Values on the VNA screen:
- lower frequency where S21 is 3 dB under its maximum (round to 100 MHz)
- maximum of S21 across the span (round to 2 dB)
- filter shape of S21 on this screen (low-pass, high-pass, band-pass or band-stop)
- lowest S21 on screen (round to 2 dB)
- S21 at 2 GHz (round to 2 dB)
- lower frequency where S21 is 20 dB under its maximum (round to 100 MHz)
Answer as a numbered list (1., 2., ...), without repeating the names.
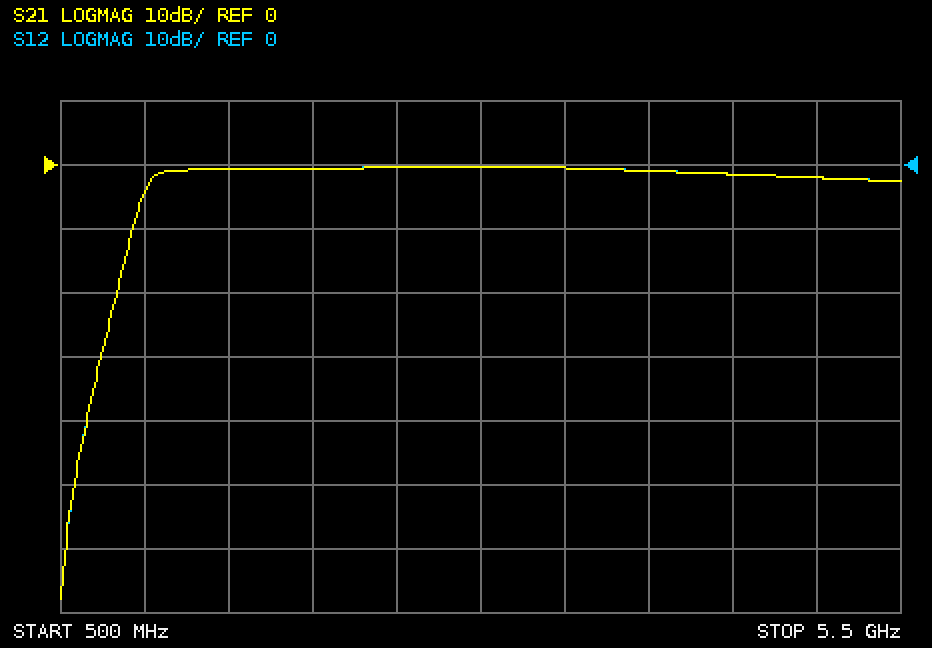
1. 1.0 GHz
2. 0 dB
3. high-pass
4. -68 dB
5. 0 dB
6. 800 MHz
